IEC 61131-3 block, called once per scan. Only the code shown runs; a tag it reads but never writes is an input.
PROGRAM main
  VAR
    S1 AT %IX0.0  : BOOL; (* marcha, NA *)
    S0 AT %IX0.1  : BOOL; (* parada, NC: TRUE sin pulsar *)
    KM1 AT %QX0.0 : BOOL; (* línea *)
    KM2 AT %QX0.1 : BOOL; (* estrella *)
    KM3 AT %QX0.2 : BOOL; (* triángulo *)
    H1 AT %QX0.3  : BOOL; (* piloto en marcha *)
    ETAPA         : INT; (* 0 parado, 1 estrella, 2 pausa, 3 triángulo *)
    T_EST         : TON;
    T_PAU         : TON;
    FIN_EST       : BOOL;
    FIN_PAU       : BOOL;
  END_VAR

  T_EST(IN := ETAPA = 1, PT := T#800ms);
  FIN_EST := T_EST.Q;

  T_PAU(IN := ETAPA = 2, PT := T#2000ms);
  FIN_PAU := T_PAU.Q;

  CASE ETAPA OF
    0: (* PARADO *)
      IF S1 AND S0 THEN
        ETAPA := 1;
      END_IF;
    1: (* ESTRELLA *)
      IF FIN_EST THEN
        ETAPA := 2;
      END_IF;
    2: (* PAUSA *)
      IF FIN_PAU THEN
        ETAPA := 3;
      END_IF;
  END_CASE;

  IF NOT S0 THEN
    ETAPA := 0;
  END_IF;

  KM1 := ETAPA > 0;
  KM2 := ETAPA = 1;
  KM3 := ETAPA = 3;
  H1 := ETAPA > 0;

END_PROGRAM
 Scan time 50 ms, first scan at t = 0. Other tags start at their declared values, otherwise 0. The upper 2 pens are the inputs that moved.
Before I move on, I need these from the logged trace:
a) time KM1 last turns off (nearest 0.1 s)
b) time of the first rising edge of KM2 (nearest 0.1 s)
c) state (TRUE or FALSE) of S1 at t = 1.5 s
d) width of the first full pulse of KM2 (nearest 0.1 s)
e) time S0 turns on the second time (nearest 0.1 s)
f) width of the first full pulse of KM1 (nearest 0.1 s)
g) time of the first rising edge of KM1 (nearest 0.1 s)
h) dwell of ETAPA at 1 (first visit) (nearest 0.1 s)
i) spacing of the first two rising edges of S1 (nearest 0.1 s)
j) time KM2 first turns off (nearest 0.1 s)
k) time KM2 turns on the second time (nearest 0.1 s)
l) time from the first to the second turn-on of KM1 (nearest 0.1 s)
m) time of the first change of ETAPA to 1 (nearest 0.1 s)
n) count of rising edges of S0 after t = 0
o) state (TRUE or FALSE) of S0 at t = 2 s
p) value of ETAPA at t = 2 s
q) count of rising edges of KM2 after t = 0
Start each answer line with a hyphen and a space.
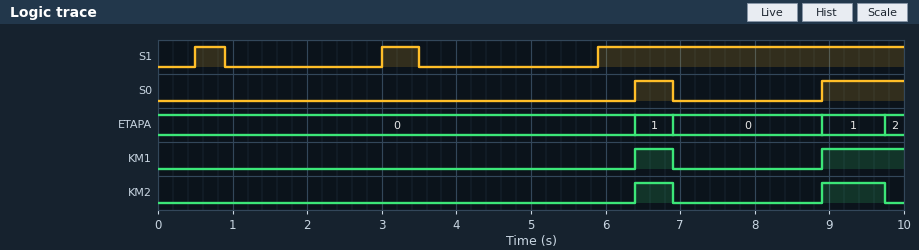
- 6.9 s
- 6.4 s
- FALSE
- 0.5 s
- 8.9 s
- 0.5 s
- 6.4 s
- 0.5 s
- 2.5 s
- 6.9 s
- 8.9 s
- 2.5 s
- 6.4 s
- 2
- FALSE
- 0
- 2
